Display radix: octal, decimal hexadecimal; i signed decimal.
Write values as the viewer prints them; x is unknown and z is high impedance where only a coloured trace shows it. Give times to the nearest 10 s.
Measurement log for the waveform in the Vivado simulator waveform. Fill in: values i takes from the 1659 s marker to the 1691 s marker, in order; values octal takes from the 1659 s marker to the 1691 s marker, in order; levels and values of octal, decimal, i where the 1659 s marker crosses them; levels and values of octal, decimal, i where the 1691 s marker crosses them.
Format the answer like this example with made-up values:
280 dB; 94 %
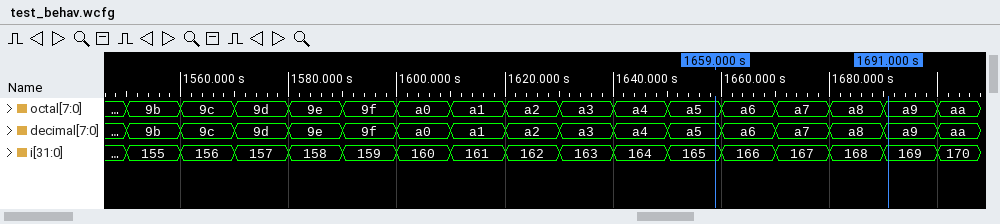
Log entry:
165, 166, 167, 168, 169; a5, a6, a7, a8, a9; octal=a5, decimal=a5, i=165; octal=a9, decimal=a9, i=169
